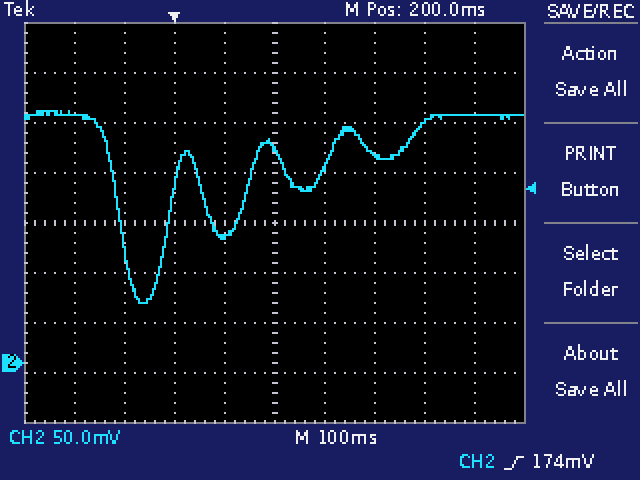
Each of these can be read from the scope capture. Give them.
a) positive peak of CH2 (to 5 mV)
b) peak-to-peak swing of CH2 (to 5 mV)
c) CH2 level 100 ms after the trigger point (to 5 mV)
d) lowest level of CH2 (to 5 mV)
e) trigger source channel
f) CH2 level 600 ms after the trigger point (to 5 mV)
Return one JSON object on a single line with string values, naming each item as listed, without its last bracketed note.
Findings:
{"positive peak of CH2": "250 mV", "peak-to-peak swing of CH2": "190 mV", "CH2 level 100 ms after the trigger point": "125 mV", "lowest level of CH2": "60 mV", "trigger source channel": "CH2", "CH2 level 600 ms after the trigger point": "250 mV"}
